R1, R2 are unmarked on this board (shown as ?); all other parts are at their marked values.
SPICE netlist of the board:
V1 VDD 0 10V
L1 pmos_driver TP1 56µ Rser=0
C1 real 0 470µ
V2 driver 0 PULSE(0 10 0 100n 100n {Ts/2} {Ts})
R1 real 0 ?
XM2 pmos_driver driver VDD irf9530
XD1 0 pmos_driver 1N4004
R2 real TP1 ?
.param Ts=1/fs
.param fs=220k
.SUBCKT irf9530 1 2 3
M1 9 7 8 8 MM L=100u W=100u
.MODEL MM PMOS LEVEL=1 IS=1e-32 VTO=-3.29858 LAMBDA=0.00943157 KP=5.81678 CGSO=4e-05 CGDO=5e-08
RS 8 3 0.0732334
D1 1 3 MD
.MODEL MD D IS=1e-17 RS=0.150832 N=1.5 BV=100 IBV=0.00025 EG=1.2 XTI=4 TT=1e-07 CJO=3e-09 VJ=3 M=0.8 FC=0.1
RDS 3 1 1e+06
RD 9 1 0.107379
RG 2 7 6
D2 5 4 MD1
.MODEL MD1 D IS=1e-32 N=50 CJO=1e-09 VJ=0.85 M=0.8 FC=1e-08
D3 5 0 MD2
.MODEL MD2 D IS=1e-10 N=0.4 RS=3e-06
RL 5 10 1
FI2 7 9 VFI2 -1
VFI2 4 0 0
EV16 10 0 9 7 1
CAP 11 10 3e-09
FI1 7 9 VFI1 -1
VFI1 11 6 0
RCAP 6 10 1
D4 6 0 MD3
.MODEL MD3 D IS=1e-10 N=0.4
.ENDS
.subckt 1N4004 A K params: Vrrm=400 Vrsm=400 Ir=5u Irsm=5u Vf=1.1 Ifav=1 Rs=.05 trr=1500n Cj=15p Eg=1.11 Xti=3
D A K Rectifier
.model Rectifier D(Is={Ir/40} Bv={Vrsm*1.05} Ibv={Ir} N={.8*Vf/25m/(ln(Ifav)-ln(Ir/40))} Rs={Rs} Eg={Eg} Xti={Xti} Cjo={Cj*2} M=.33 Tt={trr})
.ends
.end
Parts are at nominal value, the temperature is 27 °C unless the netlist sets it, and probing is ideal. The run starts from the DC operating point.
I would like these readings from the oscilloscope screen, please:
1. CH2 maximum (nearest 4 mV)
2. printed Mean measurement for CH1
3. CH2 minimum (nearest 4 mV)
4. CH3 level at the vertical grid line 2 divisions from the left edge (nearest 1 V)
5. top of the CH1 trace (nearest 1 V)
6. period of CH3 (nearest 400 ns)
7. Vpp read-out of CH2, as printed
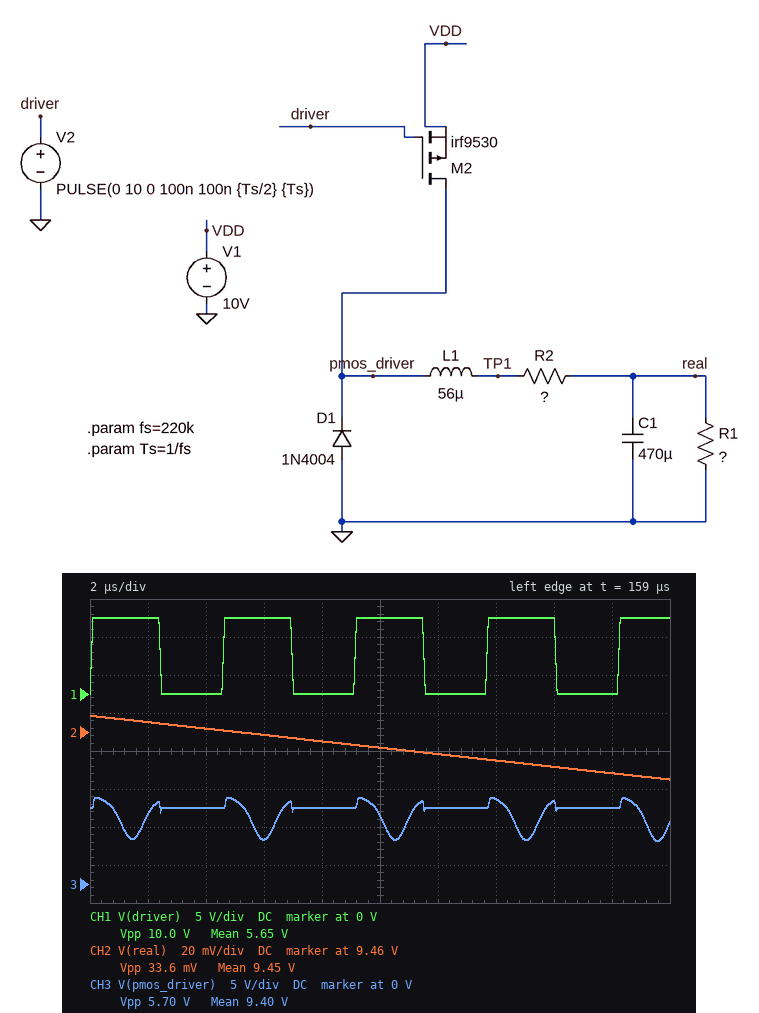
9.468 V
5.65 V
9.436 V
10 V
10 V
4.4 µs
33.6 mV
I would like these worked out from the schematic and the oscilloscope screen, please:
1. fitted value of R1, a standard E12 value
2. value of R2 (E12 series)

12 Ω
0.12 Ω
